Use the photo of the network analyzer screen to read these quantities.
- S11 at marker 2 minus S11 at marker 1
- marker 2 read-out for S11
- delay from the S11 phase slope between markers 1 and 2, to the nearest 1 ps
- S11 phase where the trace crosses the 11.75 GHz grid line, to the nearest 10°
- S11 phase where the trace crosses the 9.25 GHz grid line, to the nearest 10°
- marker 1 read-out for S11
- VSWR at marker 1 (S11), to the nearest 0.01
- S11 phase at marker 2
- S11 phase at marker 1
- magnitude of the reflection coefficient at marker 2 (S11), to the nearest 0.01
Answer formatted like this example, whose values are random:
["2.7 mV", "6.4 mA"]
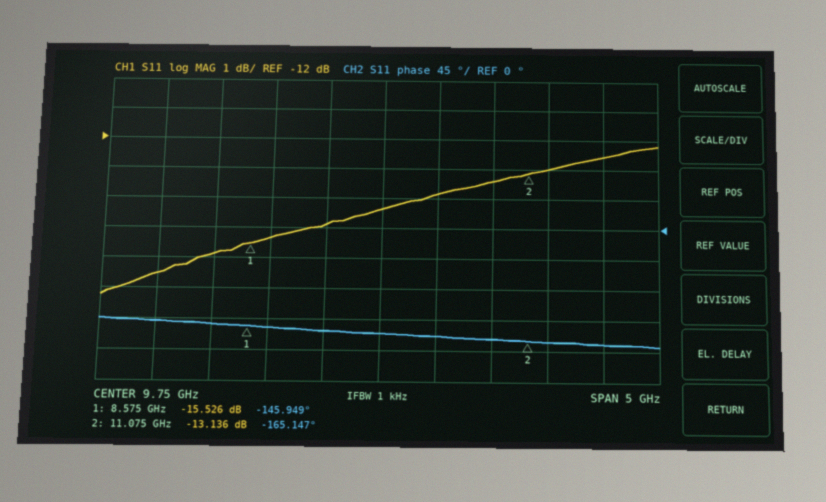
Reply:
["2.390 dB", "-13.136 dB", "21 ps", "-170°", "-150°", "-15.526 dB", "1.40", "-165.147°", "-145.949°", "0.22"]
